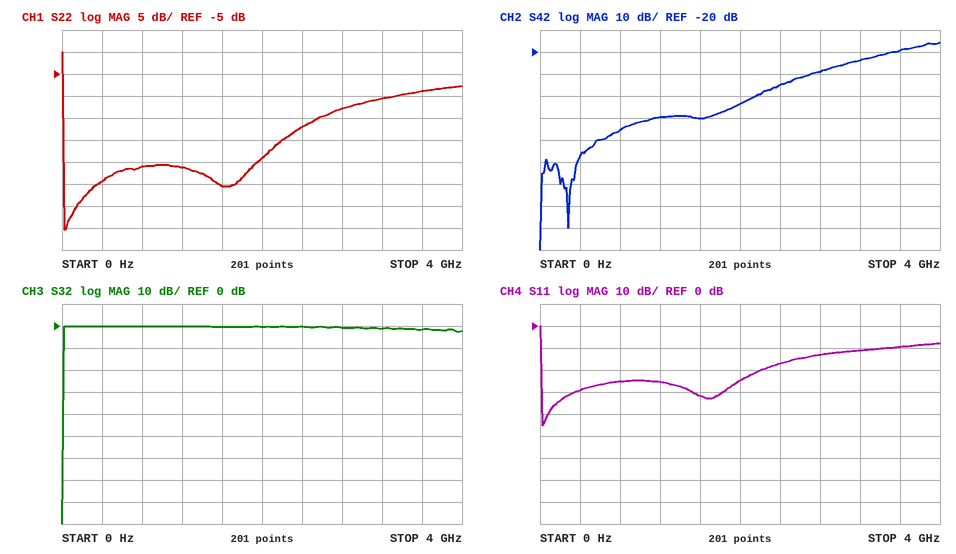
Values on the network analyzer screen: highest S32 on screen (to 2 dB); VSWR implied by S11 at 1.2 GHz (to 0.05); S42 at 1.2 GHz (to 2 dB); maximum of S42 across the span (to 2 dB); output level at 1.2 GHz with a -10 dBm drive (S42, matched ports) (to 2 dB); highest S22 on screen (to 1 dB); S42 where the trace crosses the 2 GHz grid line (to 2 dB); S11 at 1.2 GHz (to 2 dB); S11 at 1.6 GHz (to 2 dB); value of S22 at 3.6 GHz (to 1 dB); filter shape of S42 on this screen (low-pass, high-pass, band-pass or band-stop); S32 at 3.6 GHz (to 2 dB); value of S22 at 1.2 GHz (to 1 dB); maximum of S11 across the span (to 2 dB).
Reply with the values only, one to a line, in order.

0 dB
1.10
-50 dB
-16 dB
-60 dBm
0 dB
-44 dB
-26 dB
-32 dB
-9 dB
high-pass
-2 dB
-26 dB
0 dB
